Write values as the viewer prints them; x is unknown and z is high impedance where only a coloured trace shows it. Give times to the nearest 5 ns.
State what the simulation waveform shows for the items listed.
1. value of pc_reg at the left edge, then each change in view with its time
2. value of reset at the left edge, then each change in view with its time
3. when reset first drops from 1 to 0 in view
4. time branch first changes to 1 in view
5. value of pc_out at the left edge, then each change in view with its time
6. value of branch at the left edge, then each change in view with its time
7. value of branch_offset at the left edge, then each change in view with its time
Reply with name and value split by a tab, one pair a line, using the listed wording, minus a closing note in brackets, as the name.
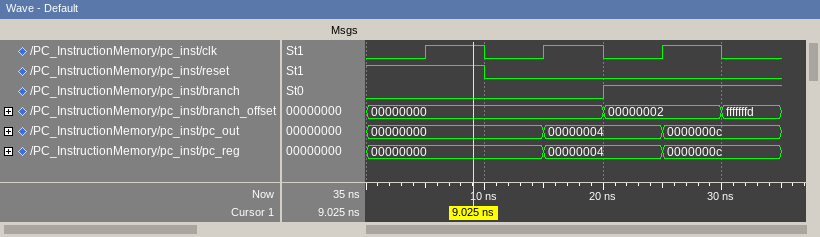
value of pc_reg at the left edge, then each change in view with its time	00000000, 00000004 at 15 ns, 0000000c at 25 ns
value of reset at the left edge, then each change in view with its time	1, 0 at 10 ns
when reset first drops from 1 to 0 in view	10 ns
time branch first changes to 1 in view	20 ns
value of pc_out at the left edge, then each change in view with its time	00000000, 00000004 at 15 ns, 0000000c at 25 ns
value of branch at the left edge, then each change in view with its time	0, 1 at 20 ns
value of branch_offset at the left edge, then each change in view with its time	00000000, 00000002 at 20 ns, fffffffd at 30 ns
